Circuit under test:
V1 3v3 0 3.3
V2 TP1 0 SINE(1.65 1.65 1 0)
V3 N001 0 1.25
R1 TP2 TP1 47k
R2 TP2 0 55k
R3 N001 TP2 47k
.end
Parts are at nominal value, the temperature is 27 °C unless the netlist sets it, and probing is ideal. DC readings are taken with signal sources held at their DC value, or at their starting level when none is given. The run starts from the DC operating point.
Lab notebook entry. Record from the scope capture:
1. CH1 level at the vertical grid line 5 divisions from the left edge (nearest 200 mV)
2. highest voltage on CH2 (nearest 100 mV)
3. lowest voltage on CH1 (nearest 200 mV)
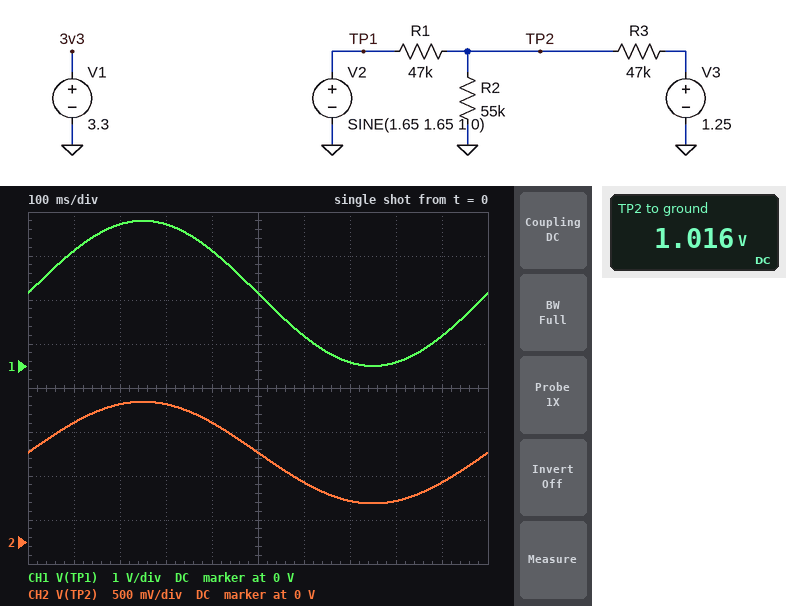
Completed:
1.6 V
1.6 V
0 V
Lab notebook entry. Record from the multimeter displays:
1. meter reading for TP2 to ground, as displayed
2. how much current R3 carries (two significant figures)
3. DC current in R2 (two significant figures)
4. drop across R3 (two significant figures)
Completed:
1.016 V
5.0 µA
18 µA
230 mV
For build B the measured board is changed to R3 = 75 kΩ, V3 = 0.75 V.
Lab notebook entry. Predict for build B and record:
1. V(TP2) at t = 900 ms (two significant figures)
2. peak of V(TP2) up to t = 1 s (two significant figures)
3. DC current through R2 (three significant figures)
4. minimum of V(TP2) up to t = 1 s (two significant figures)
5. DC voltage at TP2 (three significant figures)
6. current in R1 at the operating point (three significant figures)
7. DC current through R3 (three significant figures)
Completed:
460 mV
1.5 V
15.5 µA
190 mV
854 mV
16.9 µA
1.39 µA
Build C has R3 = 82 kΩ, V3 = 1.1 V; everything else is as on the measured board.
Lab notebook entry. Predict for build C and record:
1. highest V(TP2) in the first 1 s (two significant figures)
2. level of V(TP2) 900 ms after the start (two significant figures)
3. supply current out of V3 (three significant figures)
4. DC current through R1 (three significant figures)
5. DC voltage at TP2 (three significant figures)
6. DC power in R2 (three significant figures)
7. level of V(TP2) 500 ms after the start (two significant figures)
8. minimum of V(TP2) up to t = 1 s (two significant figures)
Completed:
1.6 V
540 mV
1.96 µA
15.1 µA
939 mV
16.0 µW
940 mV
260 mV
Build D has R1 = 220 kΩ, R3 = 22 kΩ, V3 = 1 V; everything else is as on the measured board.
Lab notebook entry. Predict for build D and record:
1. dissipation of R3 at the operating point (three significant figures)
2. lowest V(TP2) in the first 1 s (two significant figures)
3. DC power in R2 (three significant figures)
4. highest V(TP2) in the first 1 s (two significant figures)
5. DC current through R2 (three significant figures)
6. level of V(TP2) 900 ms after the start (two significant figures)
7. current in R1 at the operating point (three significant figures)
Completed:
2.27 µW
670 mV
11.0 µW
890 mV
14.1 µA
710 mV
3.97 µA
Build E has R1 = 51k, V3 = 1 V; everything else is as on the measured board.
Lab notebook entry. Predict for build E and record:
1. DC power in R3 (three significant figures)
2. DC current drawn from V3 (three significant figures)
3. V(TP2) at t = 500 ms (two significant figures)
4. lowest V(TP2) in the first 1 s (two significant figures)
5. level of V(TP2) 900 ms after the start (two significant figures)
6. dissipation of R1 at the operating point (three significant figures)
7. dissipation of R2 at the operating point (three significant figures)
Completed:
180 nW
1.96 µA
910 mV
360 mV
590 mV
10.8 µW
15.0 µW
